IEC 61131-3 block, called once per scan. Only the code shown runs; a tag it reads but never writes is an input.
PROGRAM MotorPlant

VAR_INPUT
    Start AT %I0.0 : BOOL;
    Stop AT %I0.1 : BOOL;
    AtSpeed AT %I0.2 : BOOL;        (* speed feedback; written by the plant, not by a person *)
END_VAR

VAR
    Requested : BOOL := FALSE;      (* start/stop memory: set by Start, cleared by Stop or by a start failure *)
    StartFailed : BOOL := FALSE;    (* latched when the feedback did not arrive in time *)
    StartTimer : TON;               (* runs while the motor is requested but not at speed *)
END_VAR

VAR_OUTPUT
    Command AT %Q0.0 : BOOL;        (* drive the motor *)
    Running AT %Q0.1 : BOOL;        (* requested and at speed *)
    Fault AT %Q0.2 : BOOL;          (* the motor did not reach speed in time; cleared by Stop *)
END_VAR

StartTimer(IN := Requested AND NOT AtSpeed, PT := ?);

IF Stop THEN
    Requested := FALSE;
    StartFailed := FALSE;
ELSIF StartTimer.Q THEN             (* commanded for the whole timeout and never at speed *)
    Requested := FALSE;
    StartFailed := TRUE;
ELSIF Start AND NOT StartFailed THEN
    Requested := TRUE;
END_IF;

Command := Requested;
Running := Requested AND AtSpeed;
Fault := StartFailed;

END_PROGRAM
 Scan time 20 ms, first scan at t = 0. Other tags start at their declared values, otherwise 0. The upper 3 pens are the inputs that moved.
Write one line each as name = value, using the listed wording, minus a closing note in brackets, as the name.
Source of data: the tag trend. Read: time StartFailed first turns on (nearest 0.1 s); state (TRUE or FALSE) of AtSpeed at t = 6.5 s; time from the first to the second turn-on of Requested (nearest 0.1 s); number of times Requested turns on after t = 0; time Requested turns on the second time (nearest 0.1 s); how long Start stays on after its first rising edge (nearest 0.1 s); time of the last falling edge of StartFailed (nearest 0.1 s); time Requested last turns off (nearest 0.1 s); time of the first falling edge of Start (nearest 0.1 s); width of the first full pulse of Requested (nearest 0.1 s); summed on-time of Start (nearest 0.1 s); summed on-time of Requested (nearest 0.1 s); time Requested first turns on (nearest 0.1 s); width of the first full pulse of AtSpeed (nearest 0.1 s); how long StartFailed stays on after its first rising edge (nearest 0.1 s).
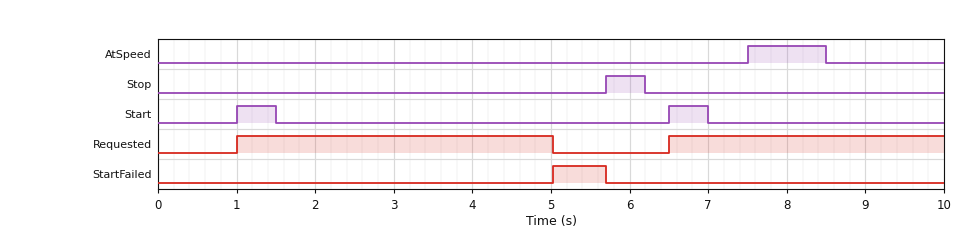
time StartFailed first turns on = 5.0 s
state (TRUE or FALSE) of AtSpeed at t = 6.5 s = FALSE
time from the first to the second turn-on of Requested = 5.5 s
number of times Requested turns on after t = 0 = 2
time Requested turns on the second time = 6.5 s
how long Start stays on after its first rising edge = 0.5 s
time of the last falling edge of StartFailed = 5.7 s
time Requested last turns off = 5.0 s
time of the first falling edge of Start = 1.5 s
width of the first full pulse of Requested = 4.0 s
summed on-time of Start = 1.0 s
summed on-time of Requested = 7.5 s
time Requested first turns on = 1.0 s
width of the first full pulse of AtSpeed = 1.0 s
how long StartFailed stays on after its first rising edge = 0.7 s
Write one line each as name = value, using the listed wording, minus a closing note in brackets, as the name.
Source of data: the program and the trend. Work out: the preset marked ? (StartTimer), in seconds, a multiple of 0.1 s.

the preset marked ? (StartTimer), in seconds, a multiple of 0.1 s = 4.0 s
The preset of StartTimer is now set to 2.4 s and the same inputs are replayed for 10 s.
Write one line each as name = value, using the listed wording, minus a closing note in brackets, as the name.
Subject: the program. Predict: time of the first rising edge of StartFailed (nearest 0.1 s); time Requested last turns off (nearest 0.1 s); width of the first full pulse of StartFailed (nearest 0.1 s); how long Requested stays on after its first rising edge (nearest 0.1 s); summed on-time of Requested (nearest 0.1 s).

time of the first rising edge of StartFailed = 3.4 s
time Requested last turns off = 3.4 s
width of the first full pulse of StartFailed = 2.3 s
how long Requested stays on after its first rising edge = 2.4 s
summed on-time of Requested = 5.9 s
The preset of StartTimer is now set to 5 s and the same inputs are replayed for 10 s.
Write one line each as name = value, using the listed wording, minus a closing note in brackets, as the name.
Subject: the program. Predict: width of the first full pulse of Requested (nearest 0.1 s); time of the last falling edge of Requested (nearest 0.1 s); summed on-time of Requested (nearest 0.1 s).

width of the first full pulse of Requested = 4.7 s
time of the last falling edge of Requested = 5.7 s
summed on-time of Requested = 8.2 s
